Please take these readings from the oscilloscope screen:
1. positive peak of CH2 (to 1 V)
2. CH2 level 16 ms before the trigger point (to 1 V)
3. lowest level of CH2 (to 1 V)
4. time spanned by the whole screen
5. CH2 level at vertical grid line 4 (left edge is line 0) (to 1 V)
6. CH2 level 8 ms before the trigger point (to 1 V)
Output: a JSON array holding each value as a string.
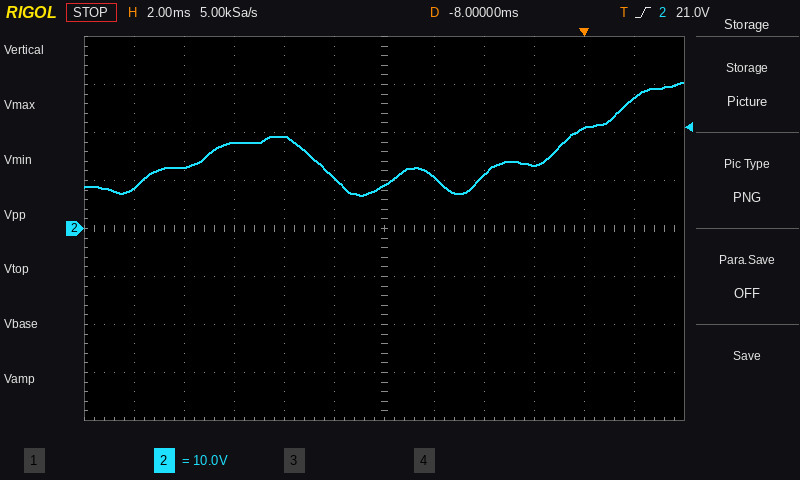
["30 V", "13 V", "7 V", "24 ms", "19 V", "9 V"]
